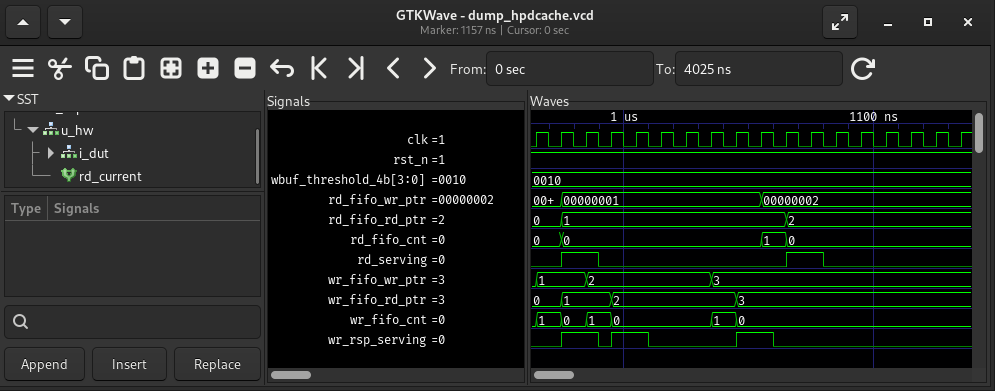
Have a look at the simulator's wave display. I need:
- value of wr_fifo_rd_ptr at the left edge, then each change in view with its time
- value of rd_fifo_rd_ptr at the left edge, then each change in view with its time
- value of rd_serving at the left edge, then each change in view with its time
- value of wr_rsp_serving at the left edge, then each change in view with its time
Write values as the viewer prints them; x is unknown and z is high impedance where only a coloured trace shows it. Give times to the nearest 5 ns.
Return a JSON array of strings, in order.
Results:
["0, 1 at 975 ns, 2 at 995 ns, 3 at 1045 ns", "0, 1 at 975 ns, 2 at 1065 ns", "0, 1 at 975 ns, 0 at 990 ns, 1 at 1065 ns, 0 at 1080 ns", "0, 1 at 975 ns, 0 at 990 ns, 1 at 995 ns, 0 at 1010 ns, 1 at 1045 ns, 0 at 1060 ns"]
